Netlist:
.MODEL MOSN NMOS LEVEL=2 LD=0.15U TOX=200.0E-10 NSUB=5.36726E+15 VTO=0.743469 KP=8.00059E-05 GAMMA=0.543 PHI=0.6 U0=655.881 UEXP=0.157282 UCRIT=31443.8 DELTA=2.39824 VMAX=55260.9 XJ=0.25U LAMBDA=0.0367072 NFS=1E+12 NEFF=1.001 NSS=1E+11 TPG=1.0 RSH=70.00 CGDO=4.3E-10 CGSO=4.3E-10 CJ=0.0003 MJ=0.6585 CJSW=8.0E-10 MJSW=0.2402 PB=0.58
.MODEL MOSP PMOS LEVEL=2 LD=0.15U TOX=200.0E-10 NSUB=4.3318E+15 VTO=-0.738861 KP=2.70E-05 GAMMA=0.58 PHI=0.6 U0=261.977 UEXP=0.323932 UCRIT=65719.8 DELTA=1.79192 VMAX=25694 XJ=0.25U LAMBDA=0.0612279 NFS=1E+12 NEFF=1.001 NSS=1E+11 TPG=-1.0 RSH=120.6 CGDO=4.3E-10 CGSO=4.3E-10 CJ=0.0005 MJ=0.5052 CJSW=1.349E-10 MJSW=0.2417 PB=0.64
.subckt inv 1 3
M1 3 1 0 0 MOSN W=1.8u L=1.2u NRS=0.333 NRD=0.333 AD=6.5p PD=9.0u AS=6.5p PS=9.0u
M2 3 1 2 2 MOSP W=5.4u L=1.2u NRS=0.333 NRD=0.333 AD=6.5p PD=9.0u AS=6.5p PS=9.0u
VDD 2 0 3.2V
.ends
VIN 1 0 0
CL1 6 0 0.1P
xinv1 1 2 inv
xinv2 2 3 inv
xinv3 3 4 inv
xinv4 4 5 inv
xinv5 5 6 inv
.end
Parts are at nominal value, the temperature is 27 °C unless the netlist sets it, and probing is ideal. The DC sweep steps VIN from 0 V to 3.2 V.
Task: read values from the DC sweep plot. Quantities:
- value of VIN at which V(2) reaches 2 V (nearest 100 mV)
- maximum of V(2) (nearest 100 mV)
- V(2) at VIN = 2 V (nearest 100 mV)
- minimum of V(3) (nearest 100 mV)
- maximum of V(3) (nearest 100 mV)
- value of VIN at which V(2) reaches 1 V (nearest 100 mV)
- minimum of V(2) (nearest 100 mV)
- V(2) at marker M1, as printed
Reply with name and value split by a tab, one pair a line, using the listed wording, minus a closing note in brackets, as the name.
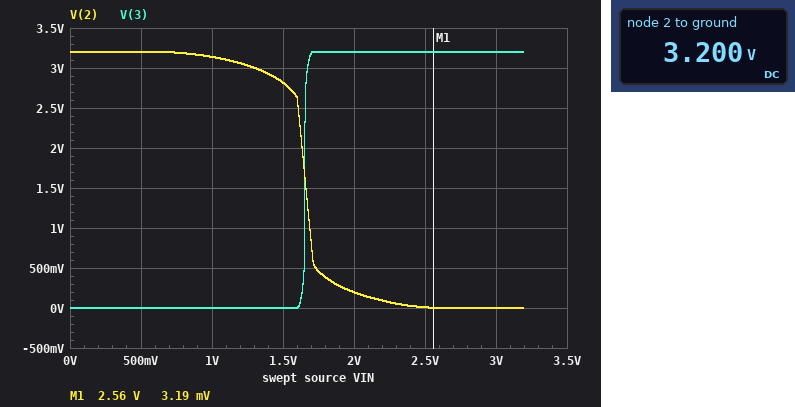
value of VIN at which V(2) reaches 2 V	1.6 V
maximum of V(2)	3.2 V
V(2) at VIN = 2 V	200 mV
minimum of V(3)	0 V
maximum of V(3)	3.2 V
value of VIN at which V(2) reaches 1 V	1.7 V
minimum of V(2)	0 V
V(2) at marker M1, as printed	3.19 mV
